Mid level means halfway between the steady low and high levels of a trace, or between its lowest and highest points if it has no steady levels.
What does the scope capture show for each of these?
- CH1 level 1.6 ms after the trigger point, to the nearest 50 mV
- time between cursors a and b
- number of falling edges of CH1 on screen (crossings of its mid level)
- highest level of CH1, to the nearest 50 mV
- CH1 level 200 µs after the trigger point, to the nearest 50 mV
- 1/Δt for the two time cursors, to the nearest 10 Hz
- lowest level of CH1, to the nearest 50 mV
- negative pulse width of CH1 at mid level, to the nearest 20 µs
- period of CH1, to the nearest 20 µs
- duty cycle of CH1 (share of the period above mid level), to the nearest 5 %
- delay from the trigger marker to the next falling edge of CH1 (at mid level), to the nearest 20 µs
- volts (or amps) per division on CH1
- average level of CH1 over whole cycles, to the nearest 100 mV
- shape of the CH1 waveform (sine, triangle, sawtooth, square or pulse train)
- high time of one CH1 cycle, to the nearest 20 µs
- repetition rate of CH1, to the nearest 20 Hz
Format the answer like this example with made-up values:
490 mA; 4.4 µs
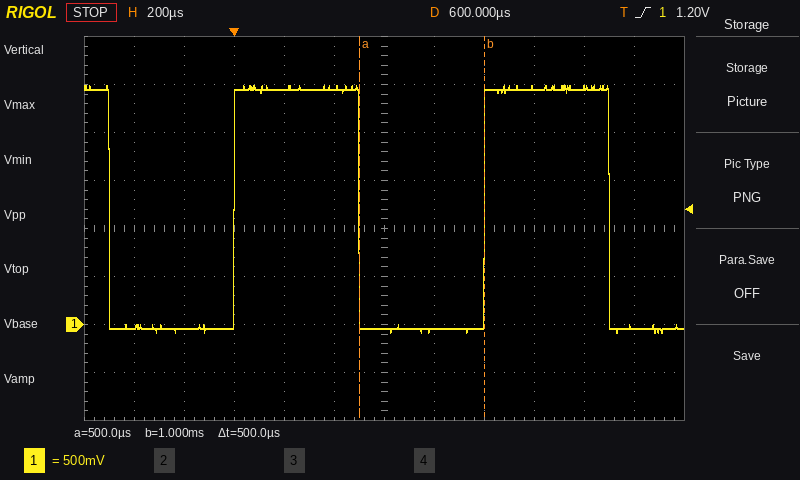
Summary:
-50 mV; 500 µs; 3; 2.50 V; 2.45 V; 2.00 kHz; -100 mV; 500 µs; 1.00 ms; 50 %; 500 µs; 500 mV; 1.2 V; square; 500 µs; 1.00 kHz
